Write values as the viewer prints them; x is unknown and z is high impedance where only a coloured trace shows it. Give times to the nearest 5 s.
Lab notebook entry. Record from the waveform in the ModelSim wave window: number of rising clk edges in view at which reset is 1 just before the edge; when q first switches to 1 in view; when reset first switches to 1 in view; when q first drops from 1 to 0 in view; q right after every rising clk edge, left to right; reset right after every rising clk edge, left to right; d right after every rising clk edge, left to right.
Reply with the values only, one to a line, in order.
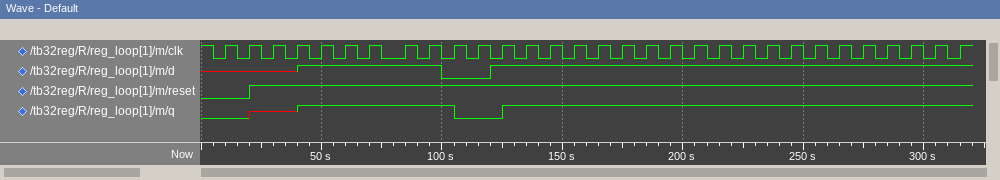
29
40 s
20 s
105 s
0 x x 1 1 1 1 1 1 0 0 1 1 1 1 1 1 1 1 1 1 1 1 1 1 1 1 1 1 1 1
0 1 1 1 1 1 1 1 1 1 1 1 1 1 1 1 1 1 1 1 1 1 1 1 1 1 1 1 1 1 1
x x x 1 1 1 1 1 1 0 0 1 1 1 1 1 1 1 1 1 1 1 1 1 1 1 1 1 1 1 1
